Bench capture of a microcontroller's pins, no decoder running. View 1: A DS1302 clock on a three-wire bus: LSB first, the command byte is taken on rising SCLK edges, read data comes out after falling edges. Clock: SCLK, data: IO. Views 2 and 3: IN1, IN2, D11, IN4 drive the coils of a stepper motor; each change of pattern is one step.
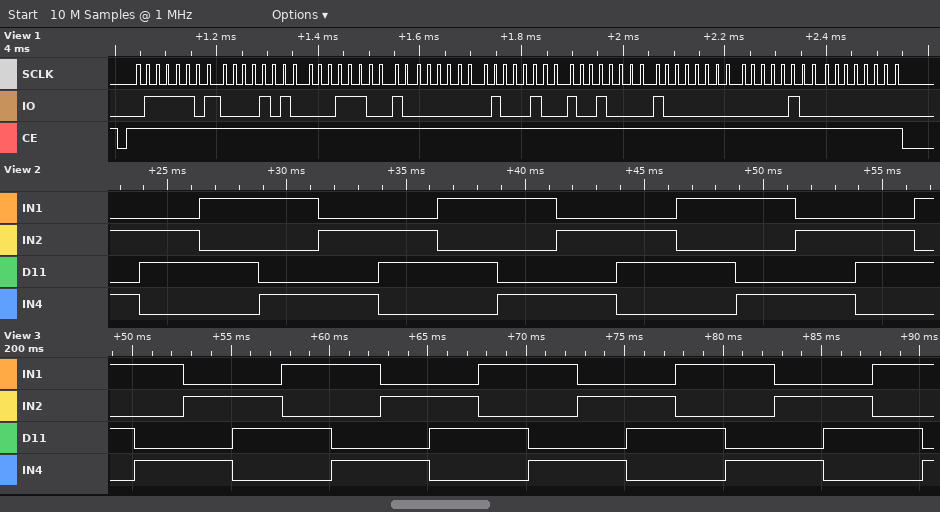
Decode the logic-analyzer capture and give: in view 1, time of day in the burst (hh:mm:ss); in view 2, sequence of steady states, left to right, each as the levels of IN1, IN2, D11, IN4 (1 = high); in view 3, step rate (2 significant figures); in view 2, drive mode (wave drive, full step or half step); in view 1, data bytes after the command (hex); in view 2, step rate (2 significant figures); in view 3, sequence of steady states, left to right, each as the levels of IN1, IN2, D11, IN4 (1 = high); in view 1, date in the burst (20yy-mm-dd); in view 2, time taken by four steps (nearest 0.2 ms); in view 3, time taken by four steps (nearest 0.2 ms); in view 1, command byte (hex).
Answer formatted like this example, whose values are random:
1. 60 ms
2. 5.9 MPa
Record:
1. 01:38:50
2. 0101 0110 1010 1001 0101 0110 1010 1001 0101 0110 1010 1001 0101 0110 1010
3. 400 steps/s
4. full step
5. 50 38 01 22 09 01 20 00
6. 400 steps/s
7. 1010 1001 0101 0110 1010 1001 0101 0110 1010 1001 0101 0110 1010 1001 0101 0110 1010 1001
8. 2020-09-22
9. 10.0 ms
10. 10.0 ms
11. 0xBE
